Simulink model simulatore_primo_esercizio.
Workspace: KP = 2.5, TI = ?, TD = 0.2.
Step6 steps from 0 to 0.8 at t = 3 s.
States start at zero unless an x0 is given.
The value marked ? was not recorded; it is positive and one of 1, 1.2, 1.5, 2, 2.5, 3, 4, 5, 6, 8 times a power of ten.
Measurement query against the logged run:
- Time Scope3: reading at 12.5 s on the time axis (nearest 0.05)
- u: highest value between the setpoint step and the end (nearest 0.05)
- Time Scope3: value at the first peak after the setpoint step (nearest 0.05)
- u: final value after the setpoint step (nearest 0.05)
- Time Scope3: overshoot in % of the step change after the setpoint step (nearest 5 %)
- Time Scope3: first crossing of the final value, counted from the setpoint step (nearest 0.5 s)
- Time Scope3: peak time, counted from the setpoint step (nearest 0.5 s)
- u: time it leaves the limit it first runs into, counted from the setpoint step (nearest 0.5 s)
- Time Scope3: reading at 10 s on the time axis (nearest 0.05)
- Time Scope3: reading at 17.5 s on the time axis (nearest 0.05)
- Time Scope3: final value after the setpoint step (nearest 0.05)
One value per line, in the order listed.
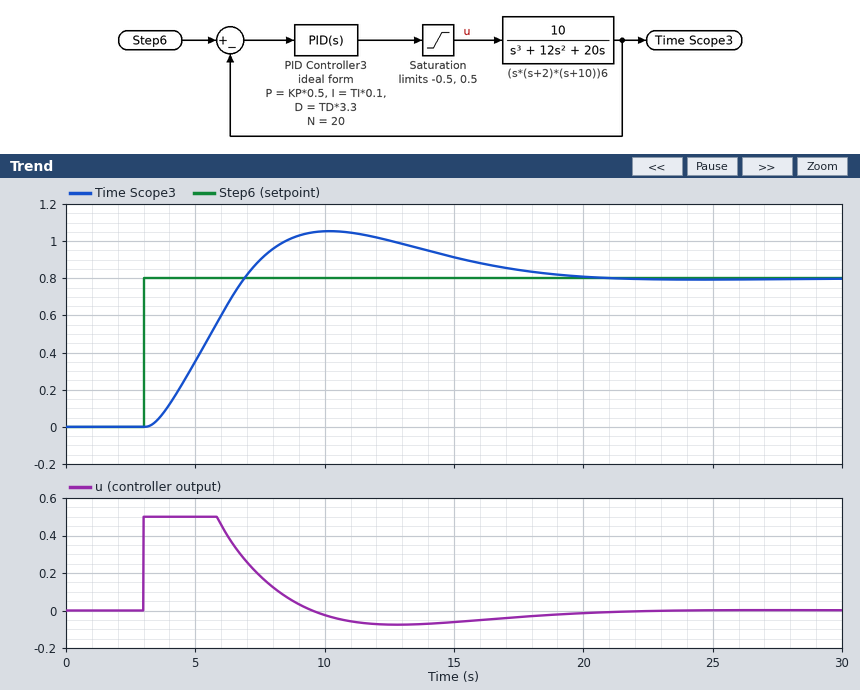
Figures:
1.00
0.50
1.05
0.00
30 %
4.0 s
7.0 s
3.0 s
1.05
0.85
0.80
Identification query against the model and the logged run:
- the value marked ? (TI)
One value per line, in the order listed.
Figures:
2
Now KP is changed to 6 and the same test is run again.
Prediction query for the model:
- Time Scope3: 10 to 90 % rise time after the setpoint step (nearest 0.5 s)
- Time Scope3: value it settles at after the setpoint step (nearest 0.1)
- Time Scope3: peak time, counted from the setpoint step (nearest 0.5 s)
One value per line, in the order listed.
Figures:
2.5 s
0.8
6.0 s
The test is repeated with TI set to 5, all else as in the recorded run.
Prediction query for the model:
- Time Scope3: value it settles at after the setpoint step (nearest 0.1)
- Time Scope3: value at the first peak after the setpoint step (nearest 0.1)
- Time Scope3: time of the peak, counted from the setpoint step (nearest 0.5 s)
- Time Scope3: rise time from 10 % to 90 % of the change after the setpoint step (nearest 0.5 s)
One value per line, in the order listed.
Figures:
0.8
1.3
6.5 s
2.5 s
